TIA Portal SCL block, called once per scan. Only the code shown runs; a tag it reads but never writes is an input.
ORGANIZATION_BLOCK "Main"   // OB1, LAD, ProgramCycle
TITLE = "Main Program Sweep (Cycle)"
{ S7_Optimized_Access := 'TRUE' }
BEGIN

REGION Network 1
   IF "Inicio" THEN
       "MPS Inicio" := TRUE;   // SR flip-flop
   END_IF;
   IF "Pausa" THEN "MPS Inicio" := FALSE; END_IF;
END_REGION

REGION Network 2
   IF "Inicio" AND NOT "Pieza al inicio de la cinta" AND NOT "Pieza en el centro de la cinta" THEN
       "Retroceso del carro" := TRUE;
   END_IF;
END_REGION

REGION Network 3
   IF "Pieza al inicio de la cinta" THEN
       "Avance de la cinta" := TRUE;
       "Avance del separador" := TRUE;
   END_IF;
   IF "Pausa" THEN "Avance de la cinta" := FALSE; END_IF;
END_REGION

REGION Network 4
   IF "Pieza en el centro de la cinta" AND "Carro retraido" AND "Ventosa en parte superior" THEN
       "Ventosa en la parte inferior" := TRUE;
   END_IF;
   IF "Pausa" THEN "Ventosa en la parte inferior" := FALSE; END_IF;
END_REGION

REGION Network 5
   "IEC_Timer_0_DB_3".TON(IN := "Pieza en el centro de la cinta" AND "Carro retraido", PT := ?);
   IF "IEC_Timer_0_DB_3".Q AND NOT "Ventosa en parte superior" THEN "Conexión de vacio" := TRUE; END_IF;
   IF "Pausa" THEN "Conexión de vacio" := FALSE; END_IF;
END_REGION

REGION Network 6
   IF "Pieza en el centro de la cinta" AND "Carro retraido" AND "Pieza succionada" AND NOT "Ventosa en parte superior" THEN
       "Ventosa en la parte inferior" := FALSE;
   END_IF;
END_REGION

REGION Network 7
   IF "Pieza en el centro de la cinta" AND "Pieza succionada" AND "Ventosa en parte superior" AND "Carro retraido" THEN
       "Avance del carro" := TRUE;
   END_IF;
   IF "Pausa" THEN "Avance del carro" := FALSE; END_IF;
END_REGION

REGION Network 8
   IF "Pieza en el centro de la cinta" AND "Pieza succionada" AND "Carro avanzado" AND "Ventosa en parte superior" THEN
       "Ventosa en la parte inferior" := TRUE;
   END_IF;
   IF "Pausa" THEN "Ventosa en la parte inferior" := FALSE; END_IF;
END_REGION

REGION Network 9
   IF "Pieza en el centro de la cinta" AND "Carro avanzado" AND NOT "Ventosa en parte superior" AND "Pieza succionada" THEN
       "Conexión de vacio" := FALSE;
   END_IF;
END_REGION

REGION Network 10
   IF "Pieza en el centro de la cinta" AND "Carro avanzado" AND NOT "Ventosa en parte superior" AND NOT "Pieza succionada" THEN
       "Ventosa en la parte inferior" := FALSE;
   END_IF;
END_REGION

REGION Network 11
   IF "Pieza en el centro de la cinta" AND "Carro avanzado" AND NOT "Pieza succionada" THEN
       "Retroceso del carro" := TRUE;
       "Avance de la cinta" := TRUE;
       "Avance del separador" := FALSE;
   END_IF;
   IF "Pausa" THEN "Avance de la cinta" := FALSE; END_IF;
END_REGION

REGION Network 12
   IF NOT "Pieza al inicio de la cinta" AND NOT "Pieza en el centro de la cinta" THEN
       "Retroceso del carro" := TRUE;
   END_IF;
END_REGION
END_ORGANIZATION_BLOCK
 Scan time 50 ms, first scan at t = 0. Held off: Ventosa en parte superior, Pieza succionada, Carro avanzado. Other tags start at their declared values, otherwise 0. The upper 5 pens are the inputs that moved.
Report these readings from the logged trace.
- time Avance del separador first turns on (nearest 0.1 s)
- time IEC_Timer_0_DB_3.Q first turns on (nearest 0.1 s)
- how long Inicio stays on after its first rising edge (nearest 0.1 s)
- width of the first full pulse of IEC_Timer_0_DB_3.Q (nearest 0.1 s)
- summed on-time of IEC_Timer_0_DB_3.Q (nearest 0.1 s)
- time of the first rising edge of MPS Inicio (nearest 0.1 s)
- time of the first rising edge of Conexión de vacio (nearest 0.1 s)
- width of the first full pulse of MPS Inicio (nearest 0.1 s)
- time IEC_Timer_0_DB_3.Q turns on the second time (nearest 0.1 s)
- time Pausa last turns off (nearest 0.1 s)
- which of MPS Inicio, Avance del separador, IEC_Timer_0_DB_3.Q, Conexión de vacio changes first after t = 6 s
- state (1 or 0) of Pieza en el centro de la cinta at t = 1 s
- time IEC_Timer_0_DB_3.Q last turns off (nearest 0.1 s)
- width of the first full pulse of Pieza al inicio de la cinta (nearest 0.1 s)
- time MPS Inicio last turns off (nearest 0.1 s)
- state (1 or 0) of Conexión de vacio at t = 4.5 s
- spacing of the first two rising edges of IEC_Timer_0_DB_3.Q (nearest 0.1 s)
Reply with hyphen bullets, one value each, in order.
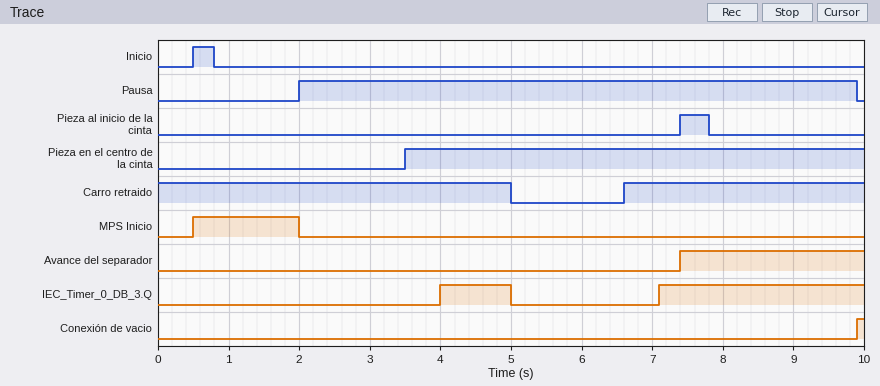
- 7.4 s
- 4.0 s
- 0.3 s
- 1.0 s
- 3.9 s
- 0.5 s
- 9.9 s
- 1.5 s
- 7.1 s
- 9.9 s
- IEC_Timer_0_DB_3.Q
- 0
- 5.0 s
- 0.4 s
- 2.0 s
- 0
- 3.1 s
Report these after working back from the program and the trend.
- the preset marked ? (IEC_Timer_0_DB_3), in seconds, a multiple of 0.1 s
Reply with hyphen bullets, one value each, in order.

- 0.5 s
